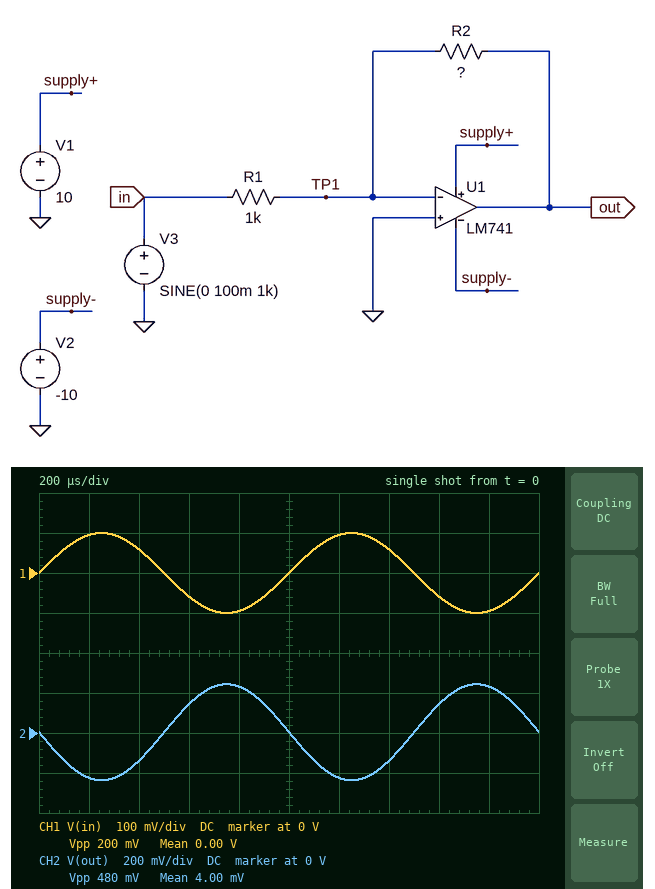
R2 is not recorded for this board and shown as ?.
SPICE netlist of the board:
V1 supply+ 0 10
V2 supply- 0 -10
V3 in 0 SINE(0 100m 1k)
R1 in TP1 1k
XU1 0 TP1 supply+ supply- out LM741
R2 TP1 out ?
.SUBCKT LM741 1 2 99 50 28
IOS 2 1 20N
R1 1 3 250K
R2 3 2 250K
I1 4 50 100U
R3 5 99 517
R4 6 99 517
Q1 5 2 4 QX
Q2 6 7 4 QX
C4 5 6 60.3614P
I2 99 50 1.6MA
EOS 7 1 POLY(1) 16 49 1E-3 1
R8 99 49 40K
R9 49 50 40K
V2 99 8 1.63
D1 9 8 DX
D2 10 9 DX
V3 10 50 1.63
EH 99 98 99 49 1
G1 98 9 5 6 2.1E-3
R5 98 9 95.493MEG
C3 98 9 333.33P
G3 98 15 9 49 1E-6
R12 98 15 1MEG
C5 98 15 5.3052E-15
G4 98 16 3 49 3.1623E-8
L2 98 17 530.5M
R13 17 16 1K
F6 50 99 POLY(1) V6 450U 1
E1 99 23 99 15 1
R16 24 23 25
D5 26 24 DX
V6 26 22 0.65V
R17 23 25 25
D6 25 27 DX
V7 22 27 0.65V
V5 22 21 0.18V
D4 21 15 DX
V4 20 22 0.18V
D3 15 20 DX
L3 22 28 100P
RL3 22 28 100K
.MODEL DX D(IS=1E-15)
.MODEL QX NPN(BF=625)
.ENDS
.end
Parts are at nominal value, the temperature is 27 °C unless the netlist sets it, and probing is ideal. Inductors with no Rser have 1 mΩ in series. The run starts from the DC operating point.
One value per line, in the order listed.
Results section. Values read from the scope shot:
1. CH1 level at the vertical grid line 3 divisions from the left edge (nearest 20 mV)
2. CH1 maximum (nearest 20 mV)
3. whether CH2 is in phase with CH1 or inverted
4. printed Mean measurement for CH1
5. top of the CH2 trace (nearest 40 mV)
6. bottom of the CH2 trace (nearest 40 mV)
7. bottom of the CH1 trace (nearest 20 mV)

-60 mV
100 mV
inverted
0.00 V
240 mV
-240 mV
-100 mV
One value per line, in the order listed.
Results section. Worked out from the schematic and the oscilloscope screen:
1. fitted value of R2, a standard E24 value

2.4 kΩ
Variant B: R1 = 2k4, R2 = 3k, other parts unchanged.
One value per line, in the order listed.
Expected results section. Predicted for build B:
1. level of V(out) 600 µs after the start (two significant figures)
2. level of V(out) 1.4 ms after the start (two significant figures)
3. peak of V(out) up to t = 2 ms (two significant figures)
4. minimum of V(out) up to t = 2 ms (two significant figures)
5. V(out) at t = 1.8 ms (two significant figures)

76 mV
-71 mV
130 mV
-120 mV
120 mV
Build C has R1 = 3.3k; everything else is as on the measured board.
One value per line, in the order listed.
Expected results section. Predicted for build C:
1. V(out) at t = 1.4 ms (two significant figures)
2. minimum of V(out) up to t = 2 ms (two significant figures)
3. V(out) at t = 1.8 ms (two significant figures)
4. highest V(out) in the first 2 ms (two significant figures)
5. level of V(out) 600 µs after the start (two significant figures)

-41 mV
-71 mV
71 mV
75 mV
45 mV
